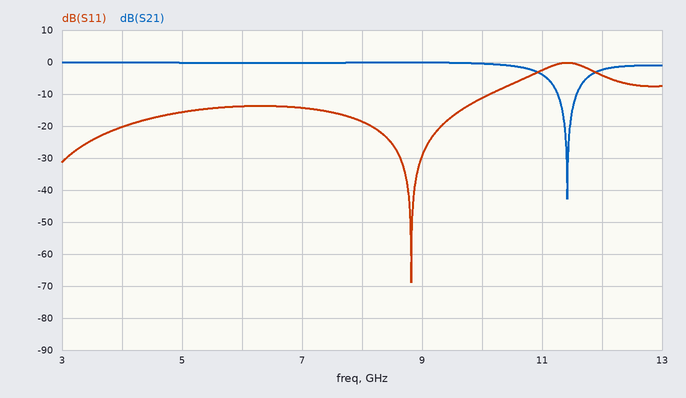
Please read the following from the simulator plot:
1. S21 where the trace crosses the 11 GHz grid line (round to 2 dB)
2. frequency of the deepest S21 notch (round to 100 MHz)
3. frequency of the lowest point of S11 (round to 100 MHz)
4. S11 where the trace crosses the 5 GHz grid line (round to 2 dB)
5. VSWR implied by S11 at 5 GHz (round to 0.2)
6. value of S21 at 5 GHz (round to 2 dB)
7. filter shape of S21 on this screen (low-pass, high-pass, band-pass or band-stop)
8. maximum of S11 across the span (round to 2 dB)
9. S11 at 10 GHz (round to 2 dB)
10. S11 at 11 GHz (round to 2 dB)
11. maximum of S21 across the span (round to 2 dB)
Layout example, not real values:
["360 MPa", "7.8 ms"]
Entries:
["-4 dB", "11.4 GHz", "8.8 GHz", "-16 dB", "1.4", "0 dB", "band-stop", "0 dB", "-12 dB", "-2 dB", "0 dB"]
